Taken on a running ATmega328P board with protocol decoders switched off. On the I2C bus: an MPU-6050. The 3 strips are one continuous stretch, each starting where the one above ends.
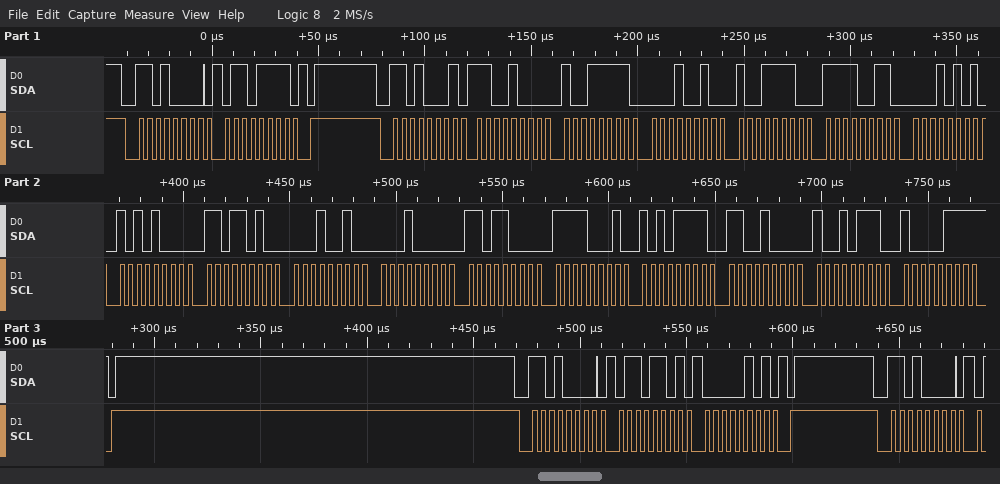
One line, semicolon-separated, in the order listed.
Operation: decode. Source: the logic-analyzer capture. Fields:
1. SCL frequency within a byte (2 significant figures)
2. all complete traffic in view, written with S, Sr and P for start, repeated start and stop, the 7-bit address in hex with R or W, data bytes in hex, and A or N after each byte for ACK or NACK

250 kHz; S 68W A 6F A P S 68R A C8 A 9F A 12 A 9E A F3 A 15 A A8 A DA A 12 A 10 A D8 A F1 A AF A C8 A 97 A 87 N P S 68W A 6D A 05 A P S 68W A
